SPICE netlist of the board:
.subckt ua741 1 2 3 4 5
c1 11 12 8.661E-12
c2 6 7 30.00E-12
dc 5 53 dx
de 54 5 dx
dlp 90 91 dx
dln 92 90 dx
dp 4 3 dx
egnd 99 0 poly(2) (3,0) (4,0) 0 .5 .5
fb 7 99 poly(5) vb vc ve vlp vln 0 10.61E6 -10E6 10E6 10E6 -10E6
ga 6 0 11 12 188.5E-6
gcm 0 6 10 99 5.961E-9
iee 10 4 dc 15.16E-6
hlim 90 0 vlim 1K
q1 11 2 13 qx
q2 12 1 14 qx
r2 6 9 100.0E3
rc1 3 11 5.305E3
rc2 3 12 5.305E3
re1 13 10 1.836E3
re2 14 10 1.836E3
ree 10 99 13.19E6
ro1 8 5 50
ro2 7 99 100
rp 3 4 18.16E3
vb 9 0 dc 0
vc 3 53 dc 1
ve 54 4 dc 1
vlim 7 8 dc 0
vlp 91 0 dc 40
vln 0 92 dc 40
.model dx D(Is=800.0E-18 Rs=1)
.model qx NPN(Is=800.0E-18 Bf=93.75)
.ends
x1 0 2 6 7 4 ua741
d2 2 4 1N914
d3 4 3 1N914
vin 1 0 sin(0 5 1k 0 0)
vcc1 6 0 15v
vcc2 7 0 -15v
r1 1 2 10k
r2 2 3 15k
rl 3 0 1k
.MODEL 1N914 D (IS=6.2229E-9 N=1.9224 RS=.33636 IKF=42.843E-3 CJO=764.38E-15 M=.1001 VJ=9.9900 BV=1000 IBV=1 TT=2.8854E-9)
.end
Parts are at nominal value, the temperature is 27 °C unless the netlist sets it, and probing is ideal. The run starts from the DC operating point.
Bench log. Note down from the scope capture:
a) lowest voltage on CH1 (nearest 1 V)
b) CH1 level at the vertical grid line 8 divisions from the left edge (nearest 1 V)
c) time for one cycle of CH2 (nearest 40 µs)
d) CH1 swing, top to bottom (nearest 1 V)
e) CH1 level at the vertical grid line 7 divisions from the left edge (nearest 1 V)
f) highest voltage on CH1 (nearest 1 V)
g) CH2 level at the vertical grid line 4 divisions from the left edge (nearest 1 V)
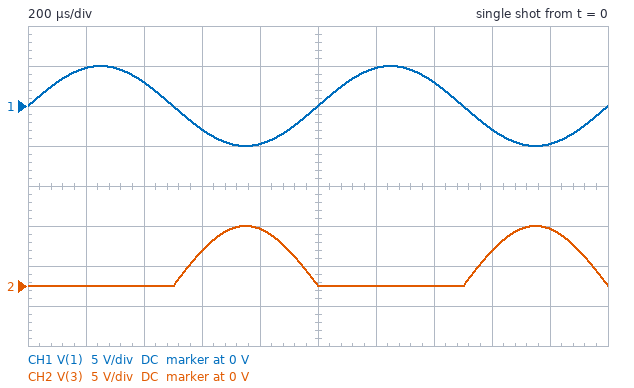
-5 V
-3 V
1.00 ms
10 V
3 V
5 V
7 V
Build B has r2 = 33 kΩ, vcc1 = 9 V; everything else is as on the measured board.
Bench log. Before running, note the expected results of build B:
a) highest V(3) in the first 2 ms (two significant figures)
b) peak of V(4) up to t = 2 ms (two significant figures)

7.9 V
8.6 V
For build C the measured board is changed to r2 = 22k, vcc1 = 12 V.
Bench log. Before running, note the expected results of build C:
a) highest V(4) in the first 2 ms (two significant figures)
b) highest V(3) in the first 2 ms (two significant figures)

12 V
11 V
